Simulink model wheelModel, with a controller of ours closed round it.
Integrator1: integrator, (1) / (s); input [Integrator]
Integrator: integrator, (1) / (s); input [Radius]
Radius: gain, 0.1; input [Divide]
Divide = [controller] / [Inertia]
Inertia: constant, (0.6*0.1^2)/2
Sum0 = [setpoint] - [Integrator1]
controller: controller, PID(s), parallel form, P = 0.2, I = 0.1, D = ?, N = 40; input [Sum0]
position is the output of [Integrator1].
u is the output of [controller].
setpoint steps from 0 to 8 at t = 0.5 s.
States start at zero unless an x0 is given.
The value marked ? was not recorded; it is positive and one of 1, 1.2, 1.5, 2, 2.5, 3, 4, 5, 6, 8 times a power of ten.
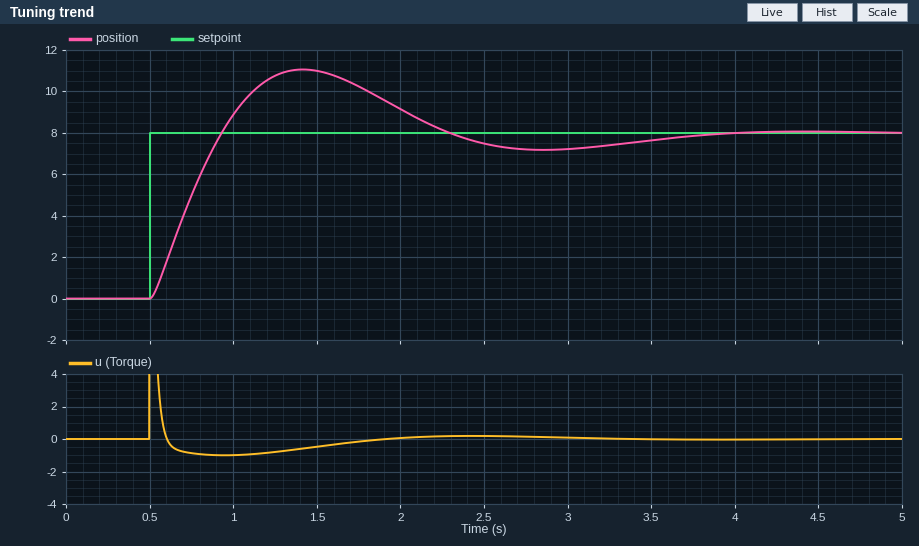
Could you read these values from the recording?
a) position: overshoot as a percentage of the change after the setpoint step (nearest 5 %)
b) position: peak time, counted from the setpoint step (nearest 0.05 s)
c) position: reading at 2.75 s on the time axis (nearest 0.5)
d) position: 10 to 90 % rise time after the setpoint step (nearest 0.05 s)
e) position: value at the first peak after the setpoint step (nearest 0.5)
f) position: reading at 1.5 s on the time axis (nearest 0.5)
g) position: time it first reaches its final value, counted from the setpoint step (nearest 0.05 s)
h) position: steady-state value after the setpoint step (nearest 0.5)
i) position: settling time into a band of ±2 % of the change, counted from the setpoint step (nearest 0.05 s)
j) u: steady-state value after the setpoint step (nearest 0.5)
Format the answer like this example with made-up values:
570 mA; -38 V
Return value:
40 %; 0.90 s; 7.0; 0.30 s; 11.0; 11.0; 0.45 s; 8.0; 3.25 s; 0.0
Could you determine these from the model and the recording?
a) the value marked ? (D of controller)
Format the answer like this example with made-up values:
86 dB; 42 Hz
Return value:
0.08
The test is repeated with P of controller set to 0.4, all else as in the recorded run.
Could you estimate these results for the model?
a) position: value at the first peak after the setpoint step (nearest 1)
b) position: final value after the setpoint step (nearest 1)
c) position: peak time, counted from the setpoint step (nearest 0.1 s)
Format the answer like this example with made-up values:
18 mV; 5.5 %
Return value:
12; 8; 0.7 s
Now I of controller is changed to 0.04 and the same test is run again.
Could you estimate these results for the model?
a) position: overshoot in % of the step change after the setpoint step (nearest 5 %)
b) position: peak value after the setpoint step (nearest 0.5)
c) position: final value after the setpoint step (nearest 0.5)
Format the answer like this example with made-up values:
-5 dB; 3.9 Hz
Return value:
35 %; 10.5; 8.0
